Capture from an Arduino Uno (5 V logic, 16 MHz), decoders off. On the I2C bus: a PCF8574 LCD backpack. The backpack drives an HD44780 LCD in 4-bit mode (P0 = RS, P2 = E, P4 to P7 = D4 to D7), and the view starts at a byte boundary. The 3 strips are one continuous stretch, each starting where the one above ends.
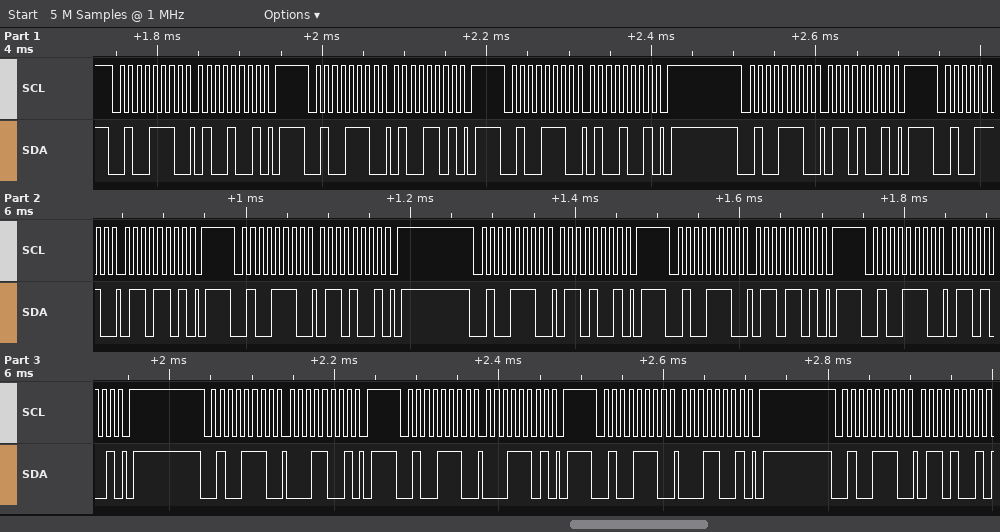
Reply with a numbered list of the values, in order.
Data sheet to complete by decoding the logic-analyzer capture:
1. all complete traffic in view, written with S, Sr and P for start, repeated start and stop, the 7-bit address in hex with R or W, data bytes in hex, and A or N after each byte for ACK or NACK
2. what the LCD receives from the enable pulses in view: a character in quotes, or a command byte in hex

1. S 27W A 49 A P S 27W A 4D A P S 27W A 49 A P S 27W A 69 A P S 27W A 6D A P S 27W A 69 A P S 27W A 69 A P S 27W A 6D A P S 27W A 69 A P S 27W A 19 A P S 27W A 1D A P S 27W A 19 A P S 27W A 69 A
2. 'F' 'a'
